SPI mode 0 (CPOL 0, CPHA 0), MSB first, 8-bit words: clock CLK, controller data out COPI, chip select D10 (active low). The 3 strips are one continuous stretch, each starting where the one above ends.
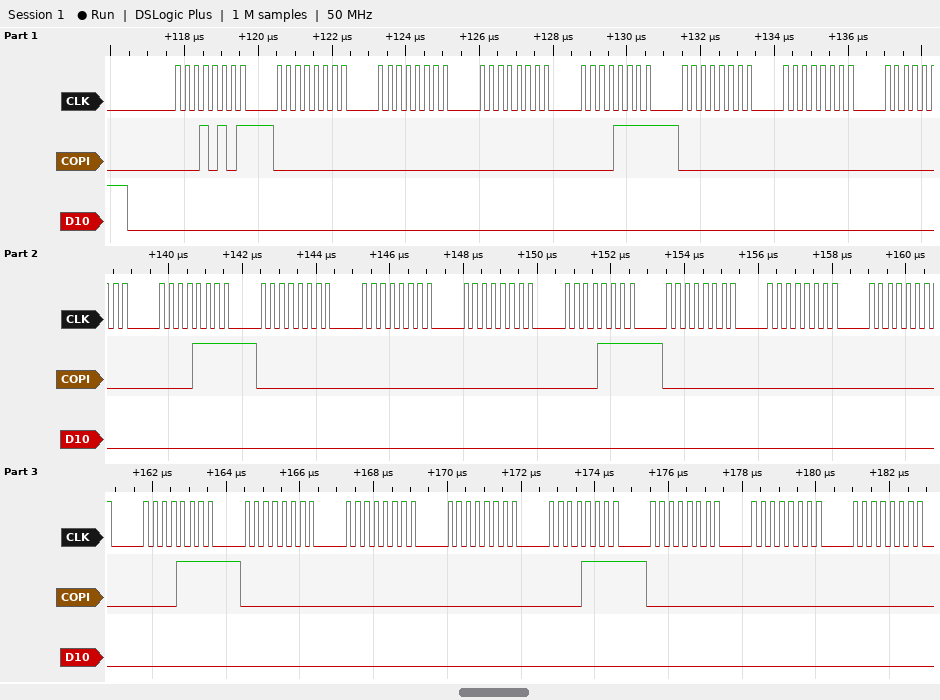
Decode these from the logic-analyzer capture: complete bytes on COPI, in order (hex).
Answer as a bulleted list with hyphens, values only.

- 15 00 00 00 0F 00 00 00 0F 00 00 00 0F 00 00 00 0F 00 00 00 0F 00 00 00
